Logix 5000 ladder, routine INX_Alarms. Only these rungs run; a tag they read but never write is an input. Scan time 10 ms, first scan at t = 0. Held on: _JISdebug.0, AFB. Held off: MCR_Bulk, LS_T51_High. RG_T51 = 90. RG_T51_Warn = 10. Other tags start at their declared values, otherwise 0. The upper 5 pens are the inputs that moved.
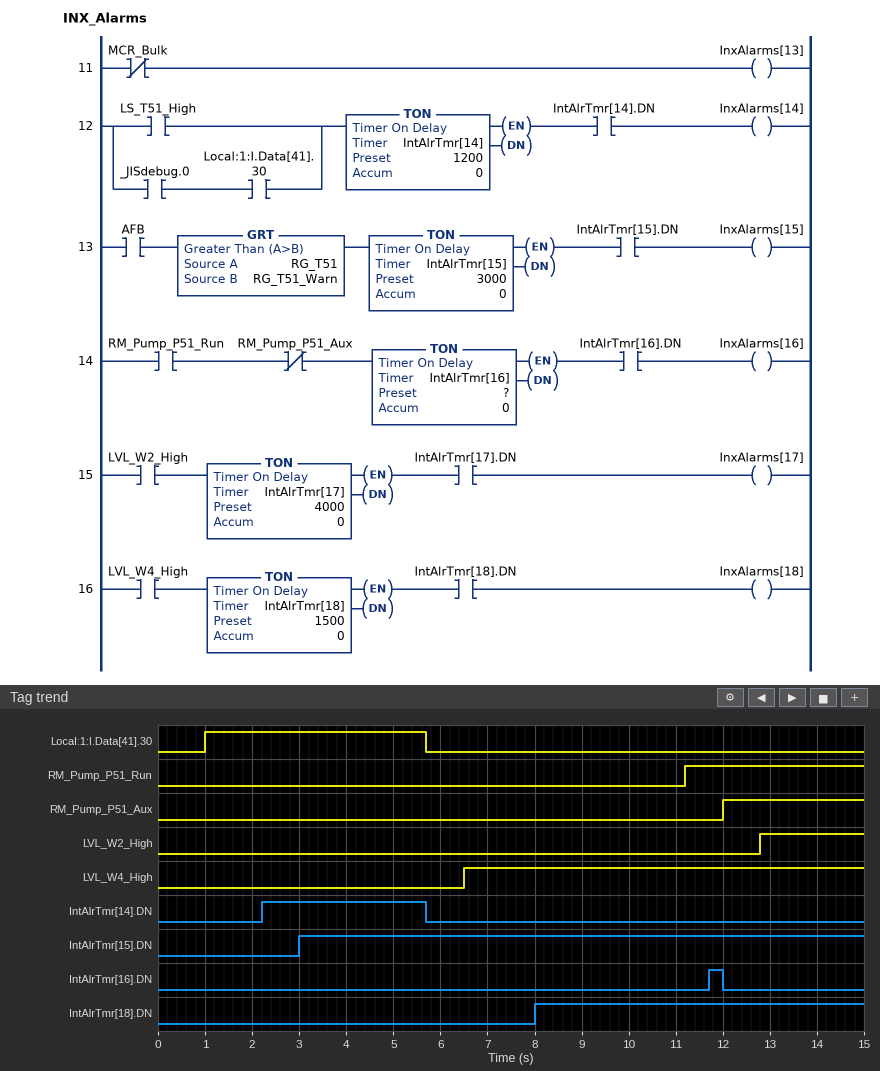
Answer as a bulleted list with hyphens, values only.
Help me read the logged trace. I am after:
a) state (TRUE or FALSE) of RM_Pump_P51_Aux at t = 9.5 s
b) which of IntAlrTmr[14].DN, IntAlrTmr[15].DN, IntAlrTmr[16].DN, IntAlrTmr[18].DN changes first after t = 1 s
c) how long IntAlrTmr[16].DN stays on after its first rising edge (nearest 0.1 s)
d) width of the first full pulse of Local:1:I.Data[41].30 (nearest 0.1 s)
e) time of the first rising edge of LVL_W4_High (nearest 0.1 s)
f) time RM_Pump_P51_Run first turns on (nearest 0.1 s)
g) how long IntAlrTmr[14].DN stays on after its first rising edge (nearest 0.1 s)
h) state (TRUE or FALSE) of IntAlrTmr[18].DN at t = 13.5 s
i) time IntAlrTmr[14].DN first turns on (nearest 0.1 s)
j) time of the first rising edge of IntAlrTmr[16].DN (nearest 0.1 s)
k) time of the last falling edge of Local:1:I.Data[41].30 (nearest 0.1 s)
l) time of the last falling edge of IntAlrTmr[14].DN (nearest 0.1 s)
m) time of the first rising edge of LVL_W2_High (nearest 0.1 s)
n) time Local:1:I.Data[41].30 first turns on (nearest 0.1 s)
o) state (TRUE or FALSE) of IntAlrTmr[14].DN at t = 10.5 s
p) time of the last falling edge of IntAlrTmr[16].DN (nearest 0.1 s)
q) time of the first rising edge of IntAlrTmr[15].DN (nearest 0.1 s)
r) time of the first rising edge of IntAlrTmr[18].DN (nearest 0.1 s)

- FALSE
- IntAlrTmr[14].DN
- 0.3 s
- 4.7 s
- 6.5 s
- 11.2 s
- 3.5 s
- TRUE
- 2.2 s
- 11.7 s
- 5.7 s
- 5.7 s
- 12.8 s
- 1.0 s
- FALSE
- 12.0 s
- 3.0 s
- 8.0 s
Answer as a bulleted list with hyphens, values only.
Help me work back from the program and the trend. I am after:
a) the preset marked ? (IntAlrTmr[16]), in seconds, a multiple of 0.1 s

- 0.5 s
